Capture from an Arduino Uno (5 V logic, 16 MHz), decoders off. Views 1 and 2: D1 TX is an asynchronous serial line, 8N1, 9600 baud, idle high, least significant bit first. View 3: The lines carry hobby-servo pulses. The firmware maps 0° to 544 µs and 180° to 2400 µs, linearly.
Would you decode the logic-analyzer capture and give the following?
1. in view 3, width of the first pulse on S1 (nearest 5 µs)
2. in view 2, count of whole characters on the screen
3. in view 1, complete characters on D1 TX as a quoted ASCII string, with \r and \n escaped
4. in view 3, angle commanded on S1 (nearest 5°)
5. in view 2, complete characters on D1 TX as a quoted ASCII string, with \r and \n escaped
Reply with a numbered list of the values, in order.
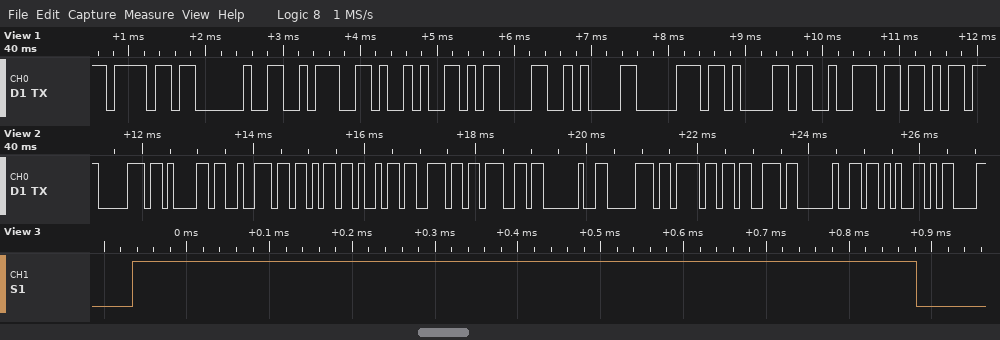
1. 945 µs
2. 14
3. "o :)\r\npark"
4. 40°
5. "parking pos +\r"
